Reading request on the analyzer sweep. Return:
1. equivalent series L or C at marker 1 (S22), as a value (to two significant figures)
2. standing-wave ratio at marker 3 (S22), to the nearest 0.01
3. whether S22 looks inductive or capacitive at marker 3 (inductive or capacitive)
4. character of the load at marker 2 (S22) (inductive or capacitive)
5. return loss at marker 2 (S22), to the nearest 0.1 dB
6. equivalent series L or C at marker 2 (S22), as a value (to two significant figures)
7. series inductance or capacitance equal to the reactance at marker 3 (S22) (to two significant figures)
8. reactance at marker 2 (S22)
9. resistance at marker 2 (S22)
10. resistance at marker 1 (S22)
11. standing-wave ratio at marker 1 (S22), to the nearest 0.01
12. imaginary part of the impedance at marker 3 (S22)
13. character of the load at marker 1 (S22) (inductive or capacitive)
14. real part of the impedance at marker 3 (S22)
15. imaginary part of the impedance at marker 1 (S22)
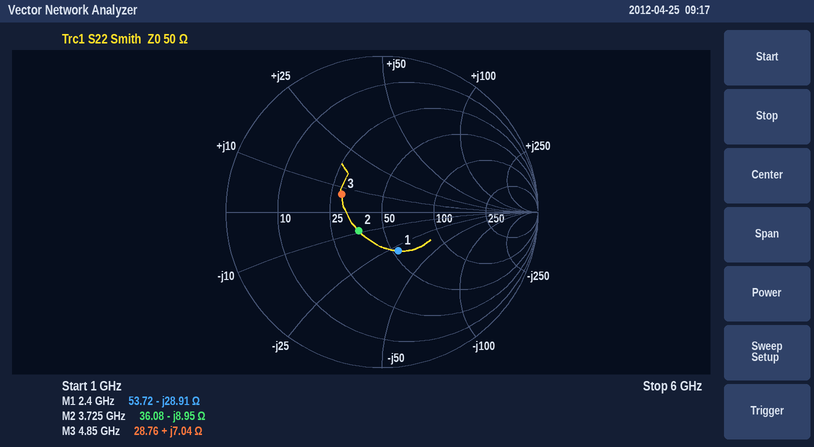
2.3 pF
1.79
inductive
capacitive
14.4 dB
4.8 pF
230 pH
-8.95 Ω
36.08 Ω
53.72 Ω
1.74
+7.04 Ω
capacitive
28.76 Ω
-28.91 Ω
